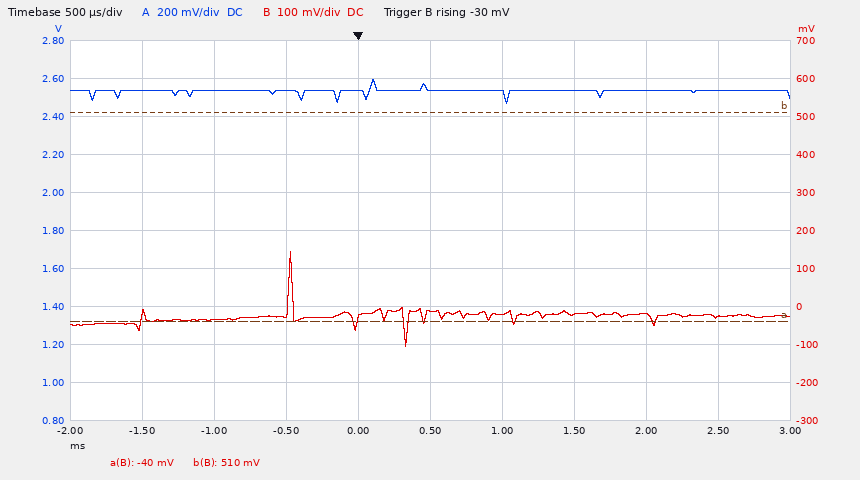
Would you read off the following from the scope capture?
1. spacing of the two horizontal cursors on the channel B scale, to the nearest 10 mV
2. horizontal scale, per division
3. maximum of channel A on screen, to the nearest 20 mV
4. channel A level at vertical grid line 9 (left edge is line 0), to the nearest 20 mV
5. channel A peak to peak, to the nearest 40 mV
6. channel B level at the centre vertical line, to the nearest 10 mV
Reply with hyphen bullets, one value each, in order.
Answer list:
- 550 mV
- 500 µs
- 2.60 V
- 2.54 V
- 120 mV
- -10 mV
